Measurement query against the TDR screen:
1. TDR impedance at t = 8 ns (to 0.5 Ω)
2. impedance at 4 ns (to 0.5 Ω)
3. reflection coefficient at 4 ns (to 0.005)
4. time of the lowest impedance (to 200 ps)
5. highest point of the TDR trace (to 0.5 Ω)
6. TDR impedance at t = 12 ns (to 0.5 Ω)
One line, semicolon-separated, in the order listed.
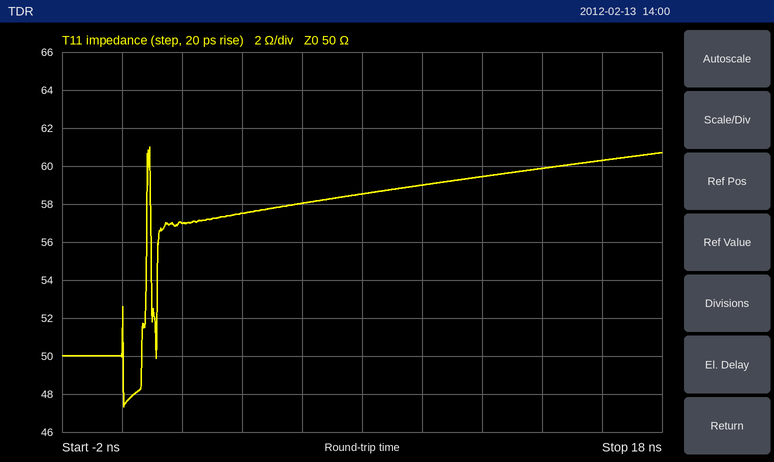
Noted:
58.5 Ω; 57.5 Ω; +0.070; 0.0 ns; 61.0 Ω; 59.5 Ω
